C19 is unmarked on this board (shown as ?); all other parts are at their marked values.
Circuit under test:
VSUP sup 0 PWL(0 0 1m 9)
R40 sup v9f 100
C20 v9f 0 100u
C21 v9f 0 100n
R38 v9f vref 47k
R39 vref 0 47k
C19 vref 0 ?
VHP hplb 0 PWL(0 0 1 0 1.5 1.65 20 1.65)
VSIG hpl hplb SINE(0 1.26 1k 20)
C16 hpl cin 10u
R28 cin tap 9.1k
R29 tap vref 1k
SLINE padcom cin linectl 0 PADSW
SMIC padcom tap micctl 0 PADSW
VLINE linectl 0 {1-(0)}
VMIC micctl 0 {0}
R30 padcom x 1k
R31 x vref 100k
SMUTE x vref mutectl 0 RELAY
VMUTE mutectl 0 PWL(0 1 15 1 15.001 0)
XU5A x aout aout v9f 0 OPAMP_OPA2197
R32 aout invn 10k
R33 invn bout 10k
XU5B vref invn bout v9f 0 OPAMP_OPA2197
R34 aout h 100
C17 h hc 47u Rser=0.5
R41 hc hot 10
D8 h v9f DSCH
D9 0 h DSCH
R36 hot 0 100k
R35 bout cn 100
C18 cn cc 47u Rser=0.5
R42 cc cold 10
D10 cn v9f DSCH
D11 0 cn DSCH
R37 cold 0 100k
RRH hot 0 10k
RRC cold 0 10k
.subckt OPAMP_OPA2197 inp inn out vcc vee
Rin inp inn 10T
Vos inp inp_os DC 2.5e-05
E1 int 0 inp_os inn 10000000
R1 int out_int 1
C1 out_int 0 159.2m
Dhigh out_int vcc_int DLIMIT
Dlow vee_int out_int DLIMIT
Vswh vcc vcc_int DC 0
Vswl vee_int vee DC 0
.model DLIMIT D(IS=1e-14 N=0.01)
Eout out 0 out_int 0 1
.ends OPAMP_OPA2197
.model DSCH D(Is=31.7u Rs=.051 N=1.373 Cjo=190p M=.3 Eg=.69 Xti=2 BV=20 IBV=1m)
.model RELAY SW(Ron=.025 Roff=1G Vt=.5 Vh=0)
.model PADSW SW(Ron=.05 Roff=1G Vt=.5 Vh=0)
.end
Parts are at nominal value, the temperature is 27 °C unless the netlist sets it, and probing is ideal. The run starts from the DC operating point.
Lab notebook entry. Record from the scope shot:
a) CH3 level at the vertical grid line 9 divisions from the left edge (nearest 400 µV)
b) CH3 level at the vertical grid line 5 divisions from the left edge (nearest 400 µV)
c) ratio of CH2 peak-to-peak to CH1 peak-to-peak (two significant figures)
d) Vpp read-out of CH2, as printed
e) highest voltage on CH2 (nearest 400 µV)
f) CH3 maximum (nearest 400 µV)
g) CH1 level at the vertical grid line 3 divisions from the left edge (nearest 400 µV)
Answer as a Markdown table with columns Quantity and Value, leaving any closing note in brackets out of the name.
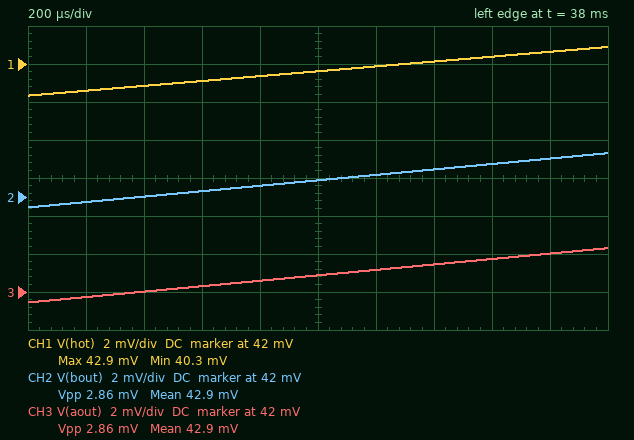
| Quantity | Value |
|---|---|
| CH3 level at the vertical grid line 9 divisions from the left edge | 44.0 mV |
| CH3 level at the vertical grid line 5 divisions from the left edge | 42.8 mV |
| ratio of CH2 peak-to-peak to CH1 peak-to-peak | 1.1 |
| Vpp read-out of CH2, as printed | 2.86 mV |
| highest voltage on CH2 | 44.4 mV |
| CH3 maximum | 44.4 mV |
| CH1 level at the vertical grid line 3 divisions from the left edge | 41.2 mV |
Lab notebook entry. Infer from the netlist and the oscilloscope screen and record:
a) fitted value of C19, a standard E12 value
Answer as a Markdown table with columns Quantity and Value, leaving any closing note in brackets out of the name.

| Quantity | Value |
|---|---|
| fitted value of C19, a standard E12 value | 120 µF |
